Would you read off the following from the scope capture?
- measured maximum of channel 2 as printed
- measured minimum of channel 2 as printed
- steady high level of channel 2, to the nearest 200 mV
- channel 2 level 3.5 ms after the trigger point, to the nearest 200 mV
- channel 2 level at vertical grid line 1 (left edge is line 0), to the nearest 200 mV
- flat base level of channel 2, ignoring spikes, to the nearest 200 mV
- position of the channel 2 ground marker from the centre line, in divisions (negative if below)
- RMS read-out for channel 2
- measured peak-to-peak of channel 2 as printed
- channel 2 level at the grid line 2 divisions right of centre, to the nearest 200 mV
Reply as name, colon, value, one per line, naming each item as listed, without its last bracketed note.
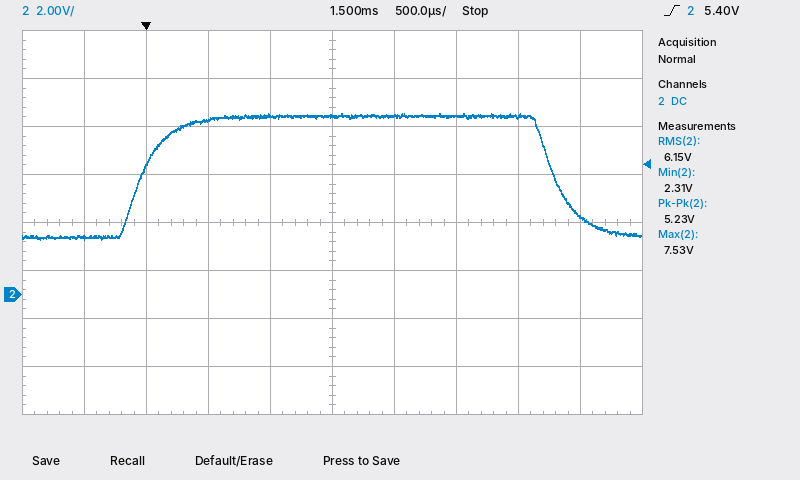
measured maximum of channel 2 as printed: 7.53 V
measured minimum of channel 2 as printed: 2.31 V
steady high level of channel 2, to the nearest 200 mV: 7.4 V
channel 2 level 3.5 ms after the trigger point, to the nearest 200 mV: 3.2 V
channel 2 level at vertical grid line 1 (left edge is line 0), to the nearest 200 mV: 2.4 V
flat base level of channel 2, ignoring spikes, to the nearest 200 mV: 2.4 V
position of the channel 2 ground marker from the centre line, in divisions: -1.5 div
RMS read-out for channel 2: 6.15 V
measured peak-to-peak of channel 2 as printed: 5.23 V
channel 2 level at the grid line 2 divisions right of centre, to the nearest 200 mV: 7.4 V
